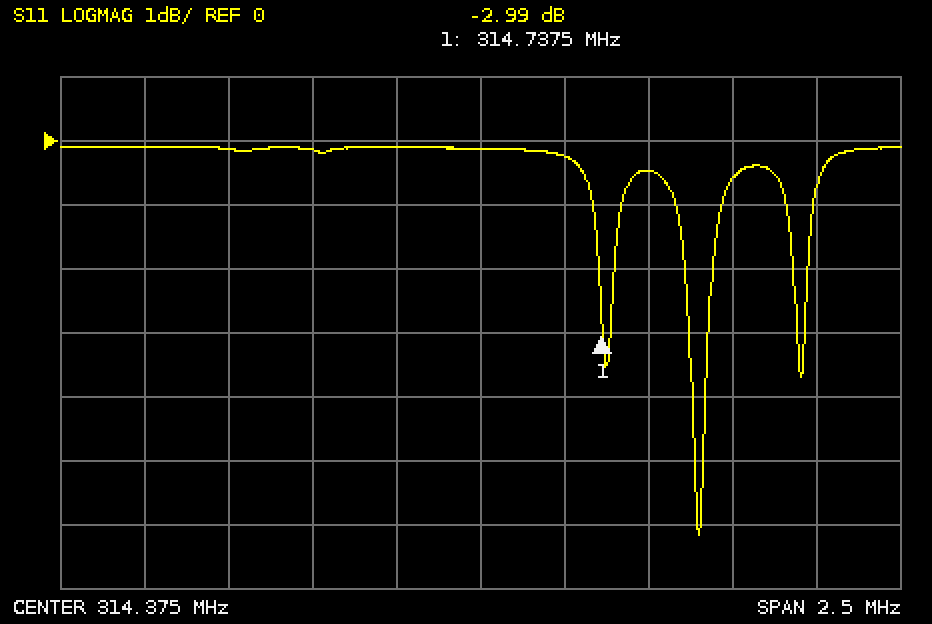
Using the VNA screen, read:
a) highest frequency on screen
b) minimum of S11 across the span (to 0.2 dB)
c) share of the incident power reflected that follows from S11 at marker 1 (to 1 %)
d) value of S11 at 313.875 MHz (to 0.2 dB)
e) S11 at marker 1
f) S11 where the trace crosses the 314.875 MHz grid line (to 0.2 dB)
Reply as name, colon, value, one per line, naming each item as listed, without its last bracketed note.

highest frequency on screen: 315.625 MHz
minimum of S11 across the span: -6.2 dB
share of the incident power reflected that follows from S11 at marker 1: 50 %
value of S11 at 313.875 MHz: -0.2 dB
S11 at marker 1: -2.99 dB
S11 where the trace crosses the 314.875 MHz grid line: -0.4 dB
